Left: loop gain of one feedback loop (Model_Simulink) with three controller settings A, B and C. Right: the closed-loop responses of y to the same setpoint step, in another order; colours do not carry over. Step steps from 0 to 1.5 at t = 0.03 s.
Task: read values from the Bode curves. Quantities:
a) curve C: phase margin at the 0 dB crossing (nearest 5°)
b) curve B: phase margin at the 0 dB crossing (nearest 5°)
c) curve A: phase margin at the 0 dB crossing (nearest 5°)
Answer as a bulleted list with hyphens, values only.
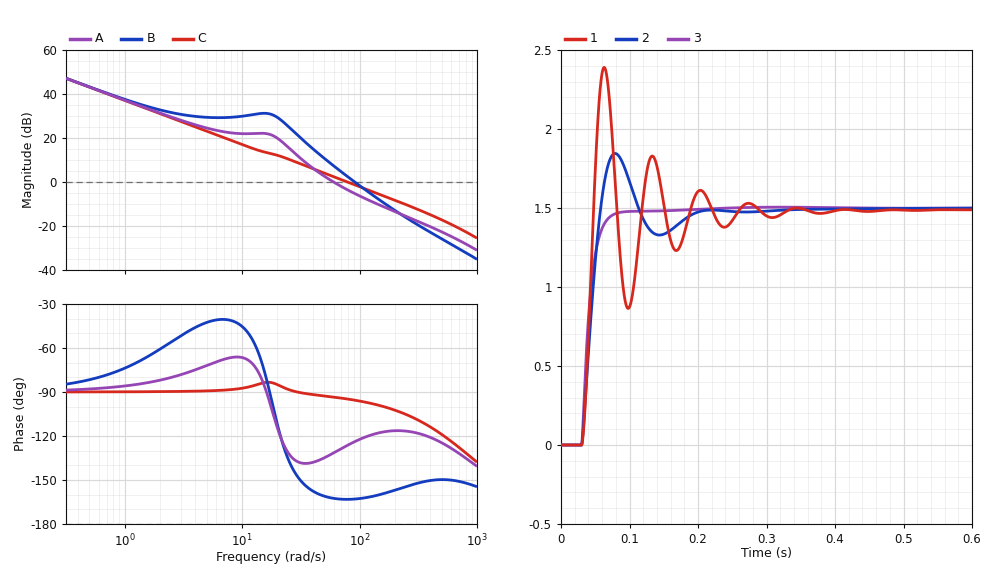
- 85°
- 15°
- 50°
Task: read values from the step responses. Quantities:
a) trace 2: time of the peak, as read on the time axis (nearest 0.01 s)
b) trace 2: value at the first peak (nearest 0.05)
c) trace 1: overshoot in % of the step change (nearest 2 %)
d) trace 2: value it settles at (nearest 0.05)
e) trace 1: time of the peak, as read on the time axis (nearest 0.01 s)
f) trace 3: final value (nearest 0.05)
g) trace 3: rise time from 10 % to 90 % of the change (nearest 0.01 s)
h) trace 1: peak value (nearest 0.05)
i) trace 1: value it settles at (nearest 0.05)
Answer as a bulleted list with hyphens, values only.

- 0.08 s
- 1.85
- 60 %
- 1.50
- 0.06 s
- 1.50
- 0.03 s
- 2.40
- 1.50
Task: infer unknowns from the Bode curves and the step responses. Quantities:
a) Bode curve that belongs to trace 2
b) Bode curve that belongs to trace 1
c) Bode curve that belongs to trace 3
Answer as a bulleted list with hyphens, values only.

- A
- B
- C
